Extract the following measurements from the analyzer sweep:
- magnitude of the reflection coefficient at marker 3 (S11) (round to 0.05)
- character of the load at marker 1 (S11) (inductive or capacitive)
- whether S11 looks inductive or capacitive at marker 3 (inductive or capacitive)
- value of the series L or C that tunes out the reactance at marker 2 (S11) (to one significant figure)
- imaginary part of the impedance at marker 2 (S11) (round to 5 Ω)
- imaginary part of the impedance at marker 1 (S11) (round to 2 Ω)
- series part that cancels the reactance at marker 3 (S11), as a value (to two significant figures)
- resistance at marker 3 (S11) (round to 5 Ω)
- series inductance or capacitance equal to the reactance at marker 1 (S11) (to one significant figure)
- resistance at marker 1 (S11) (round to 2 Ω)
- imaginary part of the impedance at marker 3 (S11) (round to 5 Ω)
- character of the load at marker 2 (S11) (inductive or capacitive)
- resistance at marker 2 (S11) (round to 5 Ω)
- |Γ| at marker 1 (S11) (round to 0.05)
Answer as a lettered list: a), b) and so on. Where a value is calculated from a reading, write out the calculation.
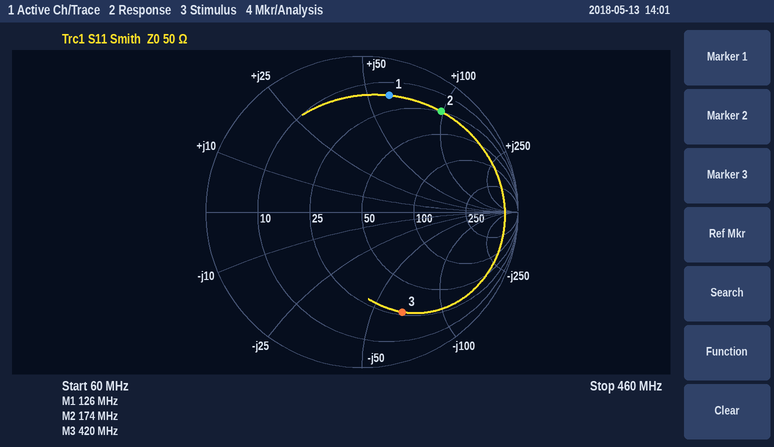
a) 0.70
b) inductive
c) capacitive
d) C = 1/(2π × 174 MHz × 100 Ω) ≈ 9 pF
e) +100 Ω
f) +60 Ω
g) L = 65 Ω/(2π × 420 MHz) ≈ 25 nH
h) 25 Ω
i) L = 60 Ω/(2π × 126 MHz) ≈ 75.8 nH, so 80 nH to one significant figure
j) 16 Ω
k) -65 Ω
l) inductive
m) 25 Ω
n) 0.75
